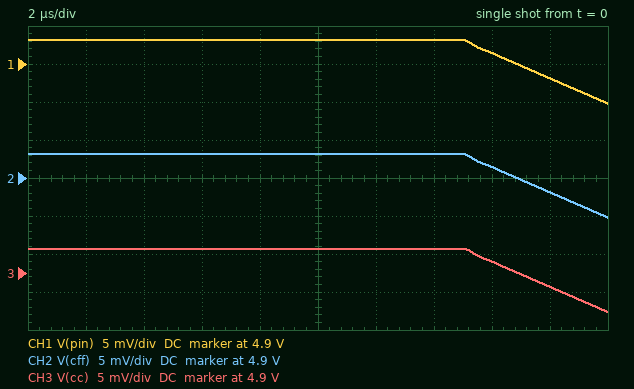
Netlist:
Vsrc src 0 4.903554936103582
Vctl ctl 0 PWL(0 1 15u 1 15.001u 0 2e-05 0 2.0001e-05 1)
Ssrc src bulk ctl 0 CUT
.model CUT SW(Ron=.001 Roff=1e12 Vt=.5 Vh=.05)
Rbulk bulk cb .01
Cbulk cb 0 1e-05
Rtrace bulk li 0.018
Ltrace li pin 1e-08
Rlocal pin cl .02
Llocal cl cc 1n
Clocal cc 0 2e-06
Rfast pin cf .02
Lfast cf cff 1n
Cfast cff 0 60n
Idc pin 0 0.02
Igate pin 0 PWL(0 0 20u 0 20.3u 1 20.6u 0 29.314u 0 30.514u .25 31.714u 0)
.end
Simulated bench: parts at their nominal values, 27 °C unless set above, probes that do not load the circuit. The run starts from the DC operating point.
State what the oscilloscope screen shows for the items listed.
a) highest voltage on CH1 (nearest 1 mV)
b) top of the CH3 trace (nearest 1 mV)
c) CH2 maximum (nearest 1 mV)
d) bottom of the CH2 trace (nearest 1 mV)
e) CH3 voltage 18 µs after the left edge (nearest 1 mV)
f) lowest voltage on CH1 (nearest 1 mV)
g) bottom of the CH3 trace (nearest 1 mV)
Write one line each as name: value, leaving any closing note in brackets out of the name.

highest voltage on CH1: 4.903 V
top of the CH3 trace: 4.903 V
CH2 maximum: 4.903 V
bottom of the CH2 trace: 4.895 V
CH3 voltage 18 µs after the left edge: 4.898 V
lowest voltage on CH1: 4.895 V
bottom of the CH3 trace: 4.895 V
